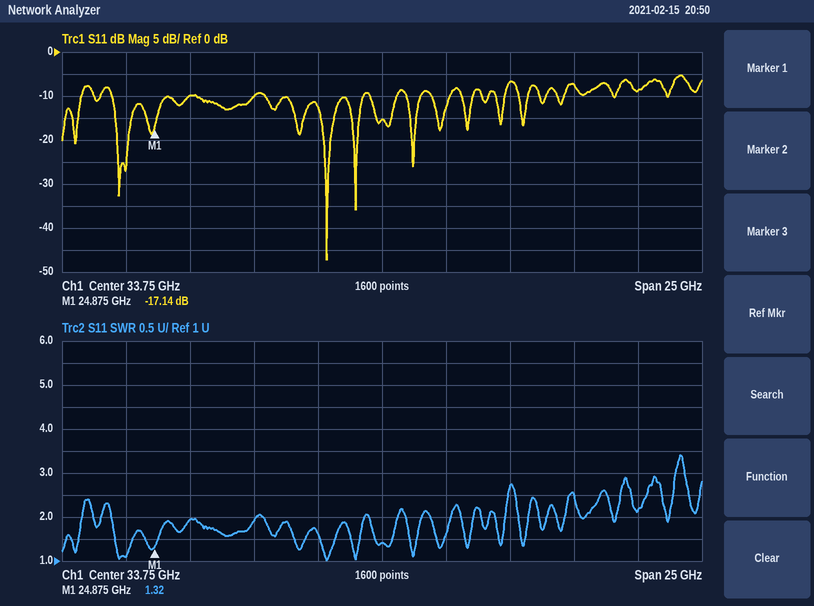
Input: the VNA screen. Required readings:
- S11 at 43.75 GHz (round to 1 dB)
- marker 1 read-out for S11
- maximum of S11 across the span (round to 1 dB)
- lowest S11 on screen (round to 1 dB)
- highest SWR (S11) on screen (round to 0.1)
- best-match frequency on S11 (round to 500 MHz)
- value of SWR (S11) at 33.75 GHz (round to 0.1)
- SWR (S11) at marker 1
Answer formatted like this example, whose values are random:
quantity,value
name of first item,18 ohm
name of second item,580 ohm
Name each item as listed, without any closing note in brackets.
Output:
quantity,value
S11 at 43.75 GHz,-9 dB
marker 1 read-out for S11,-17.14 dB
maximum of S11 across the span,-5 dB
lowest S11 on screen,-47 dB
highest SWR (S11) on screen,3.4
best-match frequency on S11,31.5 GHz
value of SWR (S11) at 33.75 GHz,1.4
SWR (S11) at marker 1,1.32
